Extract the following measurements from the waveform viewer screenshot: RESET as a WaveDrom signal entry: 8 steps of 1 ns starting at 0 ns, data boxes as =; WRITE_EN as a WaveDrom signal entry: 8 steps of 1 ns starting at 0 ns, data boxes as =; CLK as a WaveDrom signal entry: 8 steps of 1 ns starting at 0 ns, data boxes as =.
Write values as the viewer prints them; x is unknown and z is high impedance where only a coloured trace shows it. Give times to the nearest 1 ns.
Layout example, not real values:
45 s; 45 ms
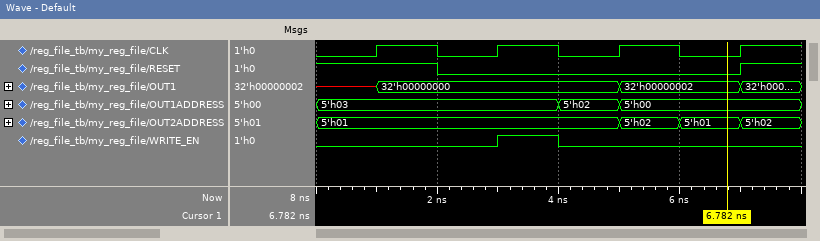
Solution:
{name: 'RESET', wave: '1.0....1'}; {name: 'WRITE_EN', wave: '0..10...'}; {name: 'CLK', wave: '01010101'}
